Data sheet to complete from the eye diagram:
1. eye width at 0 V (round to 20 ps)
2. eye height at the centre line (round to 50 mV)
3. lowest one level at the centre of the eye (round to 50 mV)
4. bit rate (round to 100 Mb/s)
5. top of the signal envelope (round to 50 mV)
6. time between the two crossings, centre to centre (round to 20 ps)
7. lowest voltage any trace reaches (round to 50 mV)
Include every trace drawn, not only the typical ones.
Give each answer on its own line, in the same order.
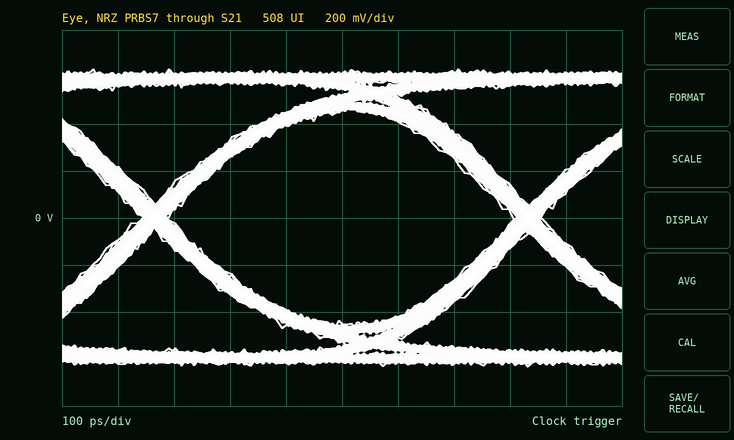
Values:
620 ps
900 mV
450 mV
1.5 Gb/s
650 mV
660 ps
-650 mV
